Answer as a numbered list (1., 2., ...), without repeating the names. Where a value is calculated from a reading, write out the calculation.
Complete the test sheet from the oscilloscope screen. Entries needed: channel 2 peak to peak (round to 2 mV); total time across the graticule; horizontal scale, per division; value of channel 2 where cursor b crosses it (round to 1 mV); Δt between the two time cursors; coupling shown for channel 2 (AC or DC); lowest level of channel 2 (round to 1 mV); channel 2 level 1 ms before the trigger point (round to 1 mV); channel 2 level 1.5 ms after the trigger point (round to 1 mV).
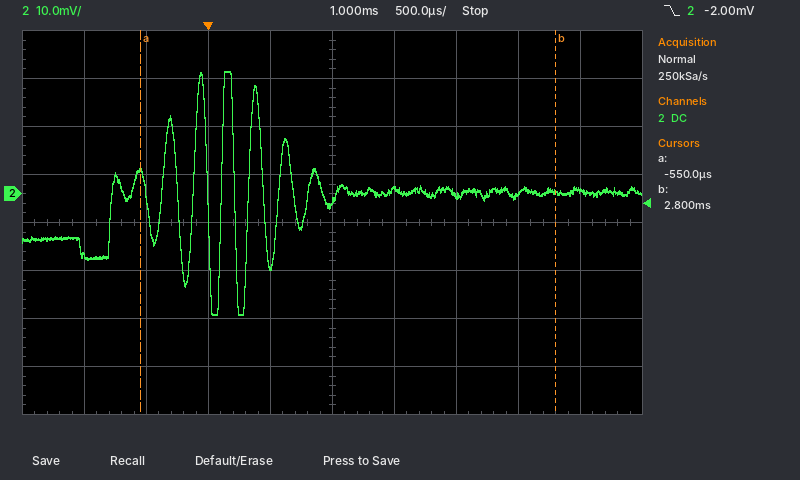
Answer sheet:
1. 50 mV
2. 5 ms
3. 500 µs
4. 0 mV
5. 2.8 ms − (-550 µs) = 3.35 ms
6. DC
7. -25 mV
8. -13 mV
9. 1 mV
